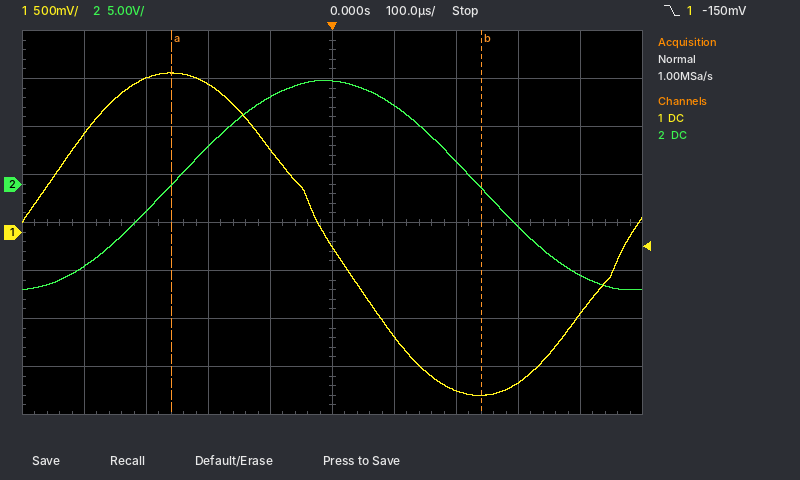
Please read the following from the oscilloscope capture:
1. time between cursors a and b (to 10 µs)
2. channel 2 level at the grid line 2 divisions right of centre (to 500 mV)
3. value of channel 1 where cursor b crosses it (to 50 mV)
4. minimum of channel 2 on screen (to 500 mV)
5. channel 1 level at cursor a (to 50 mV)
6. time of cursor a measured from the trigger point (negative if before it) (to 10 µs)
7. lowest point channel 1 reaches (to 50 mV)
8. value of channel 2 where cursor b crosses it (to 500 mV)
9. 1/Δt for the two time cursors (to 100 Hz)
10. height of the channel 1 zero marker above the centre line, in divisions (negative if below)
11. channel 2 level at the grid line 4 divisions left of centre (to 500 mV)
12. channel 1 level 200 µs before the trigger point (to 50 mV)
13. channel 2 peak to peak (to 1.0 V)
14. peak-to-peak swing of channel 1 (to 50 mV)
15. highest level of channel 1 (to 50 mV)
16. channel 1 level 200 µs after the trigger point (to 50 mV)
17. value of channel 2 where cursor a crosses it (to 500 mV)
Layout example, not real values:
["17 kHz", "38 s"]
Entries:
["500 µs", "2.5 V", "-1.70 V", "-11.0 V", "1.65 V", "-260 µs", "-1.70 V", "-500 mV", "2.0 kHz", "-0.2 div", "-8.5 V", "1.55 V", "22.0 V", "3.35 V", "1.65 V", "-1.65 V", "0.0 V"]
